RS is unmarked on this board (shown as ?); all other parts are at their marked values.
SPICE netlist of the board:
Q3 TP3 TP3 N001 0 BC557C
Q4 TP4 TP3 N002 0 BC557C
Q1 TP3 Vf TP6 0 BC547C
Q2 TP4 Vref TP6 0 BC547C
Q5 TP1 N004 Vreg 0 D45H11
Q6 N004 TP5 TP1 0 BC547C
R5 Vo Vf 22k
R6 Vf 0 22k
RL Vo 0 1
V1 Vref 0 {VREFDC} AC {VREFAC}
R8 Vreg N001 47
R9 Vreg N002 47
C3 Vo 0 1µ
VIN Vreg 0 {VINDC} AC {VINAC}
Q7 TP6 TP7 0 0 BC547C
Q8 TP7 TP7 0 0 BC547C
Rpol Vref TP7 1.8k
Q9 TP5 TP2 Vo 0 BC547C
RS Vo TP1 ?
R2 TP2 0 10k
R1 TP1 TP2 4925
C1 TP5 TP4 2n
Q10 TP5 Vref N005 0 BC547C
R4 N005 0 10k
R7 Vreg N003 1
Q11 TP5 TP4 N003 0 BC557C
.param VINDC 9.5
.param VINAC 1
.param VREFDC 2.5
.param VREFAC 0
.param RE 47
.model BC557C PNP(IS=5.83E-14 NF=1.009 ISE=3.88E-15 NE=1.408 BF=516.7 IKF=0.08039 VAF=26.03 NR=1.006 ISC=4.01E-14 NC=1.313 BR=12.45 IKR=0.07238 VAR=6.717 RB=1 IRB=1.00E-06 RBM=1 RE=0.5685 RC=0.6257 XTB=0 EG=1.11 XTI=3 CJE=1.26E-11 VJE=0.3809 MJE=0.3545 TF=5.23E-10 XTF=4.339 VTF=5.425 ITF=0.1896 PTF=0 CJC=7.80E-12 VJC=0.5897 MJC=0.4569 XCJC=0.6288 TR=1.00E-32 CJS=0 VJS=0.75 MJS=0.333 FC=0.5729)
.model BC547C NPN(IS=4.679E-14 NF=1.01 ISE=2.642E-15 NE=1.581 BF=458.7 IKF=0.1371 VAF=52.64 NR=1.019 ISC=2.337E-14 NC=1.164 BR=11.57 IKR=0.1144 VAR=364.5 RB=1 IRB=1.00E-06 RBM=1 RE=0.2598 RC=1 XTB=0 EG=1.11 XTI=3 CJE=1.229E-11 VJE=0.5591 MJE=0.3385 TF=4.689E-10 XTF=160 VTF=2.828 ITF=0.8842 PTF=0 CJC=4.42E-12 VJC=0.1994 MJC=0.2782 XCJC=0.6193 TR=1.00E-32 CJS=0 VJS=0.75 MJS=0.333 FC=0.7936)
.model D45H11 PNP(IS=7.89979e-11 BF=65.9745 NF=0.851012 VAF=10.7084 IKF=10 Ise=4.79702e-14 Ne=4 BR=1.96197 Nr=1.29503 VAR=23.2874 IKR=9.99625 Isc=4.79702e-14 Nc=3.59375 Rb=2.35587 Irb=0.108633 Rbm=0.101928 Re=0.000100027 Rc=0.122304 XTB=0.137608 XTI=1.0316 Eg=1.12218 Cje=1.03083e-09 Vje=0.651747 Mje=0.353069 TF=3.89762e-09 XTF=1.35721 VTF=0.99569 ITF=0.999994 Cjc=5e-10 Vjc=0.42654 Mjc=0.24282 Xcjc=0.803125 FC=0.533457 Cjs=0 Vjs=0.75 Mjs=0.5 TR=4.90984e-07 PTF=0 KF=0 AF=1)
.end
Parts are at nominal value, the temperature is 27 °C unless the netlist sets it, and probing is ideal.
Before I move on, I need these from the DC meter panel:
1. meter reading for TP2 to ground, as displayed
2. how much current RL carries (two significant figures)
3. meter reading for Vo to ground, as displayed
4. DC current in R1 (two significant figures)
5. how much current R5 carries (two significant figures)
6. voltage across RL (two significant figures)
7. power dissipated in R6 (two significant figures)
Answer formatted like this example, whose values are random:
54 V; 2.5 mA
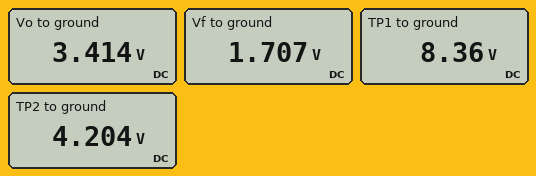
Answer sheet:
4.204 V; 3.4 A; 3.414 V; 840 µA; 78 µA; 3.4 V; 130 µW
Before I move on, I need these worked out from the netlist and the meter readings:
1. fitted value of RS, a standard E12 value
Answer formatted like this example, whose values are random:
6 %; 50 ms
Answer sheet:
1.5 Ω
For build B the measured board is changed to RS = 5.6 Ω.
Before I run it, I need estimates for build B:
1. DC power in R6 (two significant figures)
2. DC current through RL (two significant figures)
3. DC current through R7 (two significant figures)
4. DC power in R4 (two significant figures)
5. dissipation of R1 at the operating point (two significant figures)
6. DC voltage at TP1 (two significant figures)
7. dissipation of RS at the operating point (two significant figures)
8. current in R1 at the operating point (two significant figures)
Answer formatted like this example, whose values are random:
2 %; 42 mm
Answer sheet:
13 µW; 1.1 A; 160 mA; 370 µW; 3.7 mW; 6.2 V; 4.6 W; 870 µA
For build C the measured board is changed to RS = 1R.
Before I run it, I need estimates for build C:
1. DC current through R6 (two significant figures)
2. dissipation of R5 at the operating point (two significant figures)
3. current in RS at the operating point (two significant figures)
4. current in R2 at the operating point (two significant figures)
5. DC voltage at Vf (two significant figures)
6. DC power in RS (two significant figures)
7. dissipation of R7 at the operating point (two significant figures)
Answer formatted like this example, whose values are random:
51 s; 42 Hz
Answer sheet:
97 µA; 210 µW; 4.2 A; 500 µA; 2.1 V; 18 W; 4.7 mW
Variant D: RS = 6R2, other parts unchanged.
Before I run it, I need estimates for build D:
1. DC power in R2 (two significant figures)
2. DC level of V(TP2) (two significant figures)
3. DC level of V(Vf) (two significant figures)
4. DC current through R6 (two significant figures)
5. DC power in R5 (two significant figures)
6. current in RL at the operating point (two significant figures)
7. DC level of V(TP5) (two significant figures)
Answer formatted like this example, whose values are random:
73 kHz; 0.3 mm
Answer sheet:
320 µW; 1.8 V; 490 mV; 22 µA; 11 µW; 980 mA; 6.7 V
